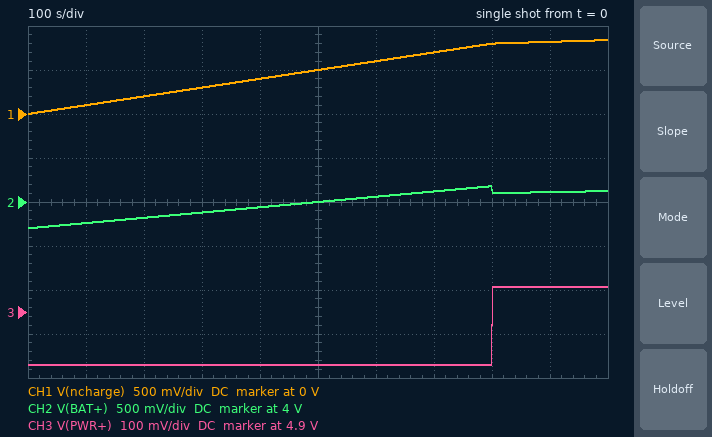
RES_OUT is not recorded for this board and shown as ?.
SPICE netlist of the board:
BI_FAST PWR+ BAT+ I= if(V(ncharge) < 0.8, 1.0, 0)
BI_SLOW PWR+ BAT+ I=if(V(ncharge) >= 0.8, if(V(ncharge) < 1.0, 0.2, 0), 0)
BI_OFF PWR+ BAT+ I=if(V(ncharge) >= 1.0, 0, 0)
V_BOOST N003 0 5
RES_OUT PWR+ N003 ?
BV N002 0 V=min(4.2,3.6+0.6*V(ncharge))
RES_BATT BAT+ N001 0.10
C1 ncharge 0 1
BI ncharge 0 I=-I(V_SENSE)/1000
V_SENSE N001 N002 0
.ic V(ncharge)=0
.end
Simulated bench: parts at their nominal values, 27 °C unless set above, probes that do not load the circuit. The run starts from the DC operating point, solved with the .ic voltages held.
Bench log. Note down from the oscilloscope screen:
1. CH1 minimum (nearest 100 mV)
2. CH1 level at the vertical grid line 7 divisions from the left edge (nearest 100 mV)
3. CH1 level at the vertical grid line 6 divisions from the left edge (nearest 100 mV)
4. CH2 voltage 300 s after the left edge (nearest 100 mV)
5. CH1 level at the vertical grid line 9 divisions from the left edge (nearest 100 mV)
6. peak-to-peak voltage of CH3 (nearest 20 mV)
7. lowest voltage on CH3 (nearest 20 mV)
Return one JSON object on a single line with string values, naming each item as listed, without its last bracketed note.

{"CH1 minimum": "0 V", "CH1 level at the vertical grid line 7 divisions from the left edge": "700 mV", "CH1 level at the vertical grid line 6 divisions from the left edge": "600 mV", "CH2 voltage 300 s after the left edge": "3.9 V", "CH1 level at the vertical grid line 9 divisions from the left edge": "800 mV", "peak-to-peak voltage of CH3": "180 mV", "lowest voltage on CH3": "4.78 V"}
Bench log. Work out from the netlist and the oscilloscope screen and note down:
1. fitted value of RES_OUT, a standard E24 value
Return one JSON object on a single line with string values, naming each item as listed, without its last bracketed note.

{"fitted value of RES_OUT, a standard E24 value": "0.22 Ω"}
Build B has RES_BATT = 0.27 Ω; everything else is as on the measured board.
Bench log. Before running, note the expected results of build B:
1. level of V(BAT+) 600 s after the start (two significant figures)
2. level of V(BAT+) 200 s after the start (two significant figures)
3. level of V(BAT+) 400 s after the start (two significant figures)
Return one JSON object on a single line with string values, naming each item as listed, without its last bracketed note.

{"level of V(BAT+) 600 s after the start": "4.2 V", "level of V(BAT+) 200 s after the start": "4.0 V", "level of V(BAT+) 400 s after the start": "4.1 V"}
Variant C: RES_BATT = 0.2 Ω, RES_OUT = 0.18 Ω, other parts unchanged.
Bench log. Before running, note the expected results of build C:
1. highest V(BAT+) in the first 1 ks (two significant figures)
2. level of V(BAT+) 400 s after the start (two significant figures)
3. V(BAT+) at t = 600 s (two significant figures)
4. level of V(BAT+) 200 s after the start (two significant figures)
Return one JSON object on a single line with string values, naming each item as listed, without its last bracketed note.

{"highest V(BAT+) in the first 1 ks": "4.3 V", "level of V(BAT+) 400 s after the start": "4.0 V", "V(BAT+) at t = 600 s": "4.2 V", "level of V(BAT+) 200 s after the start": "3.9 V"}
